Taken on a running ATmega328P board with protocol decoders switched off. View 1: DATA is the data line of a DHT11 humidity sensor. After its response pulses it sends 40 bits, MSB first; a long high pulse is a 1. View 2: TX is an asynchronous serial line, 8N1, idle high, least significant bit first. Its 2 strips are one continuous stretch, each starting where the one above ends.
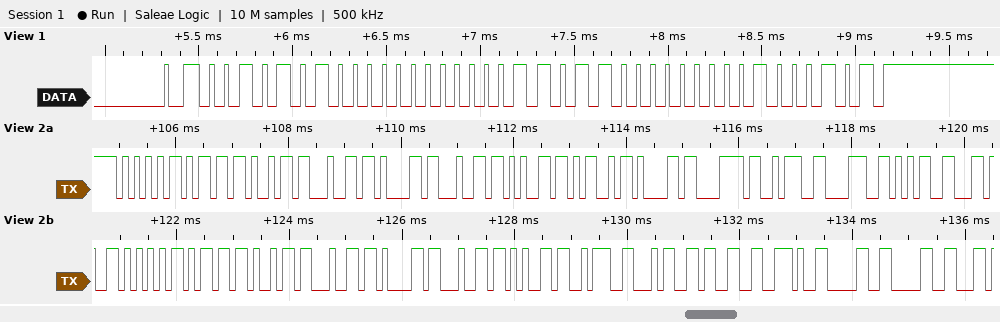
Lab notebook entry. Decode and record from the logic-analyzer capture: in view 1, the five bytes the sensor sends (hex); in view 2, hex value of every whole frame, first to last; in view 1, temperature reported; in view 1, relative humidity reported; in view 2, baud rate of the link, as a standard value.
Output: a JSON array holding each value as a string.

["2A 00 1B 00 45", "55 6D 69 64 61 64 65 4D 61 78 3A 38 35 2C 55 6D 69 64 61 64 65 3A 34 33 2E 30 30", "27.0 °C", "42 %", "9600 baud"]
